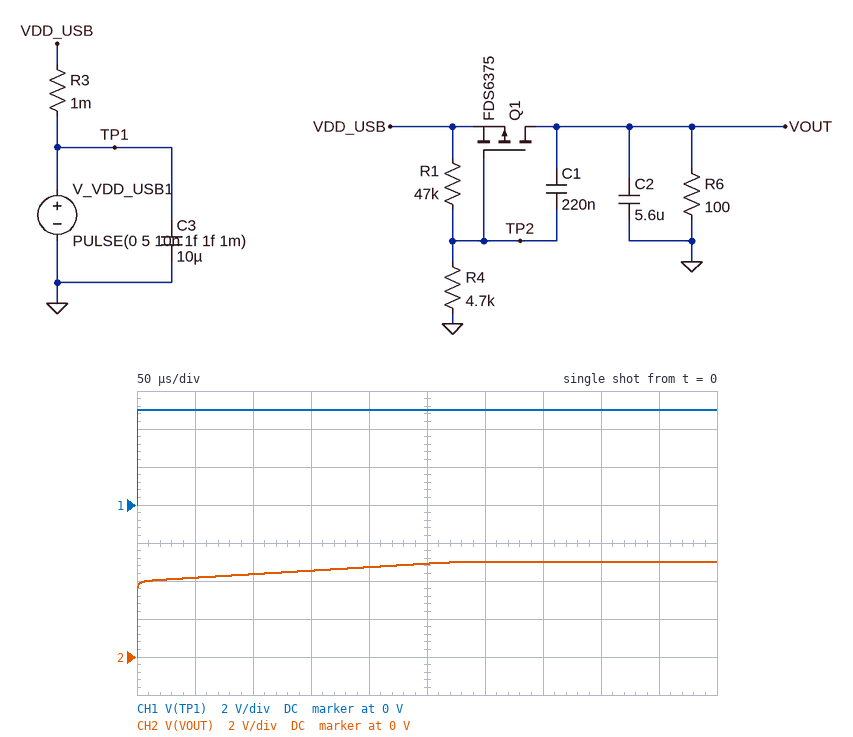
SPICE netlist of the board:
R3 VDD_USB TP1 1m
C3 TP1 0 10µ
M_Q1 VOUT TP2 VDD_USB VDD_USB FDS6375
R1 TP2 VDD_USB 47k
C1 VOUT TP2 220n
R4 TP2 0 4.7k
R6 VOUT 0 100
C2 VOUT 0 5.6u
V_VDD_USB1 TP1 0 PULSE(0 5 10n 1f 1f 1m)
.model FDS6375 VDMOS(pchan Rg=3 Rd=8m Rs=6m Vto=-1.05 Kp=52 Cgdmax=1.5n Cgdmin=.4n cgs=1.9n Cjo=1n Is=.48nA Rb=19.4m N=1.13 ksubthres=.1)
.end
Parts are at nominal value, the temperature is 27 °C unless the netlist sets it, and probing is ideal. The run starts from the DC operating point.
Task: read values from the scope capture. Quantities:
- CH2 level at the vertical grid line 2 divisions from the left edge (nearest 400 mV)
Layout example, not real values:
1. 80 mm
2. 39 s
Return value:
1. 4.4 V
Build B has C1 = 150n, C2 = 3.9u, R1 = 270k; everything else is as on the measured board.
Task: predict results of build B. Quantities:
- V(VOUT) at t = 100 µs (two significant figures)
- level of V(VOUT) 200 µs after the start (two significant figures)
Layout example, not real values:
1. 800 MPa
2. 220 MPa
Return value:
1. 4.5 V
2. 5.0 V
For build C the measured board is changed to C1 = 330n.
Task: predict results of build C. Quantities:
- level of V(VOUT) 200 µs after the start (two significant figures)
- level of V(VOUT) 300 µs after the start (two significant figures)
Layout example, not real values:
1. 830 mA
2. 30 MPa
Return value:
1. 4.5 V
2. 4.7 V
